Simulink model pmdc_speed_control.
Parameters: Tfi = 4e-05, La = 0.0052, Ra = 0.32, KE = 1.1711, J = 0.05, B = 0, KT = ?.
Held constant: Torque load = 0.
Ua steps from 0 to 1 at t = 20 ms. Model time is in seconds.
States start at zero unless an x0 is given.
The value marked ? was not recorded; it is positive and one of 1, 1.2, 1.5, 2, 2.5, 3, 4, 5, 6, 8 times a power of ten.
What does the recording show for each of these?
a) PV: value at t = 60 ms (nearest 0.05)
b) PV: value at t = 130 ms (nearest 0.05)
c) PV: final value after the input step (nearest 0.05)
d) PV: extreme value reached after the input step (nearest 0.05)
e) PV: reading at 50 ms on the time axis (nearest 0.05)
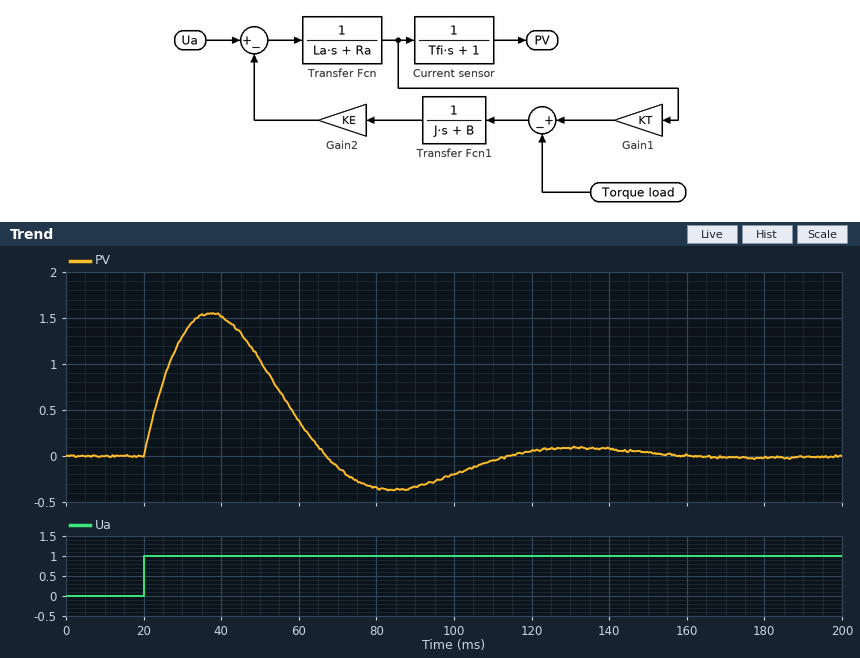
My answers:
0.40
0.10
0.00
1.55
1.05
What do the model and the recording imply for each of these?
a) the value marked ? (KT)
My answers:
1.2
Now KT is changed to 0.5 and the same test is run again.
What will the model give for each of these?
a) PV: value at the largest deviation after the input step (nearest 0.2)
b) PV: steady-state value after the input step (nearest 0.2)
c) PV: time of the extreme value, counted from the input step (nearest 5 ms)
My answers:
2.0
0.0
25 ms
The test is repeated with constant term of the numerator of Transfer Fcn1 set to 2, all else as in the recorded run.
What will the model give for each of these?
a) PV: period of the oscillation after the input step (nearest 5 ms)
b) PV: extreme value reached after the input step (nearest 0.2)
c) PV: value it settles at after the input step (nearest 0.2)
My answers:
65 ms
1.2
0.0
